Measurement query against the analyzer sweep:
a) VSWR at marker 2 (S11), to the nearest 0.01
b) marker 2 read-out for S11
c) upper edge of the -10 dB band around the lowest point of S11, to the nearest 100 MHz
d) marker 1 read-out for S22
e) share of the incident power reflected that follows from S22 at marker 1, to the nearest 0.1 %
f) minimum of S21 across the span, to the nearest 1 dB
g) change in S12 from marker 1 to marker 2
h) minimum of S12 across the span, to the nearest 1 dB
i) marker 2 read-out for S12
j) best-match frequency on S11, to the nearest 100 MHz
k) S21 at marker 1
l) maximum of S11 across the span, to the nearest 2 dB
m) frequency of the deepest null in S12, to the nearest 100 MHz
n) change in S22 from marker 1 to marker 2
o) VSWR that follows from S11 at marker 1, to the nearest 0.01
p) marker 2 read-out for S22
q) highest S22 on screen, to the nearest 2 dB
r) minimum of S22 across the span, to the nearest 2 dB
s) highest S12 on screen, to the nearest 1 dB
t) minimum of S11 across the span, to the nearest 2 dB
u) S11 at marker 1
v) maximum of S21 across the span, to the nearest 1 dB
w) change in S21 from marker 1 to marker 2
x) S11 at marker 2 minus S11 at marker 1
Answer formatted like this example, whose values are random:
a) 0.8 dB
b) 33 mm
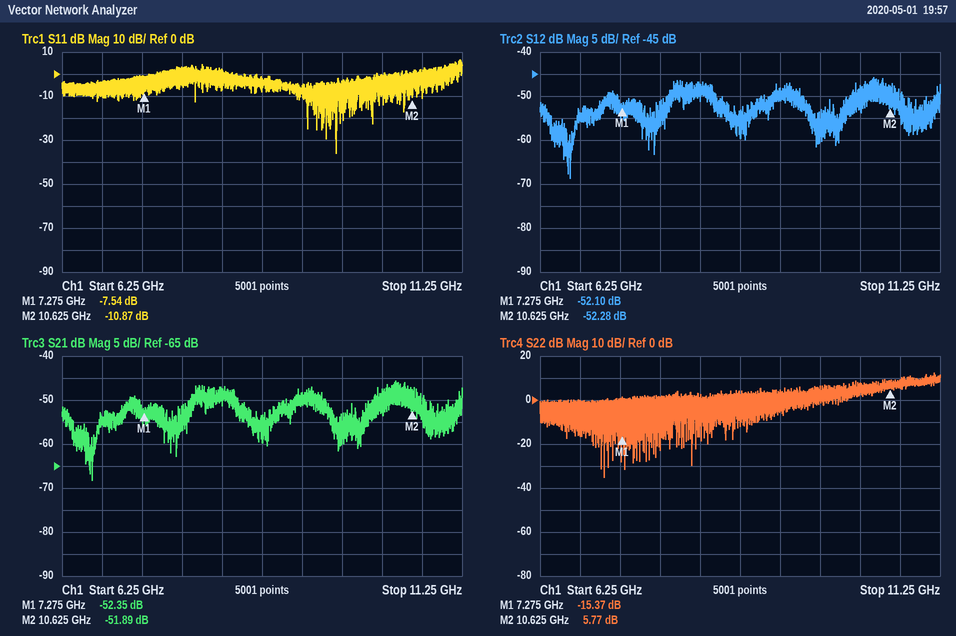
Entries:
a) 1.80
b) -10.87 dB
c) 9.7 GHz
d) -15.37 dB
e) 2.9 %
f) -68 dB
g) -0.18 dB
h) -69 dB
i) -52.28 dB
j) 9.7 GHz
k) -52.35 dB
l) 6 dB
m) 6.6 GHz
n) 21.14 dB
o) 2.45
p) 5.77 dB
q) 12 dB
r) -36 dB
s) -46 dB
t) -36 dB
u) -7.54 dB
v) -46 dB
w) 0.46 dB
x) -3.33 dB
